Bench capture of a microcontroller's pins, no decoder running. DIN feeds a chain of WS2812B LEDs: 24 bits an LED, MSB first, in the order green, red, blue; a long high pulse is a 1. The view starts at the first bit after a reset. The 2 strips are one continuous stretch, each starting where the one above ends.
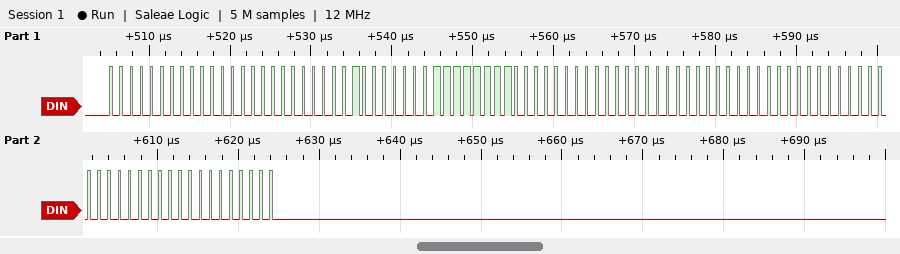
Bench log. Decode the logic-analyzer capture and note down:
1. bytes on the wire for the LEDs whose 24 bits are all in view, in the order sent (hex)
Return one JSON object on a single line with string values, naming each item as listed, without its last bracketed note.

{"bytes on the wire for the LEDs whose 24 bits are all in view, in the order sent": "00 00 00 80 FF 00 00 00 00 00 00 00"}
